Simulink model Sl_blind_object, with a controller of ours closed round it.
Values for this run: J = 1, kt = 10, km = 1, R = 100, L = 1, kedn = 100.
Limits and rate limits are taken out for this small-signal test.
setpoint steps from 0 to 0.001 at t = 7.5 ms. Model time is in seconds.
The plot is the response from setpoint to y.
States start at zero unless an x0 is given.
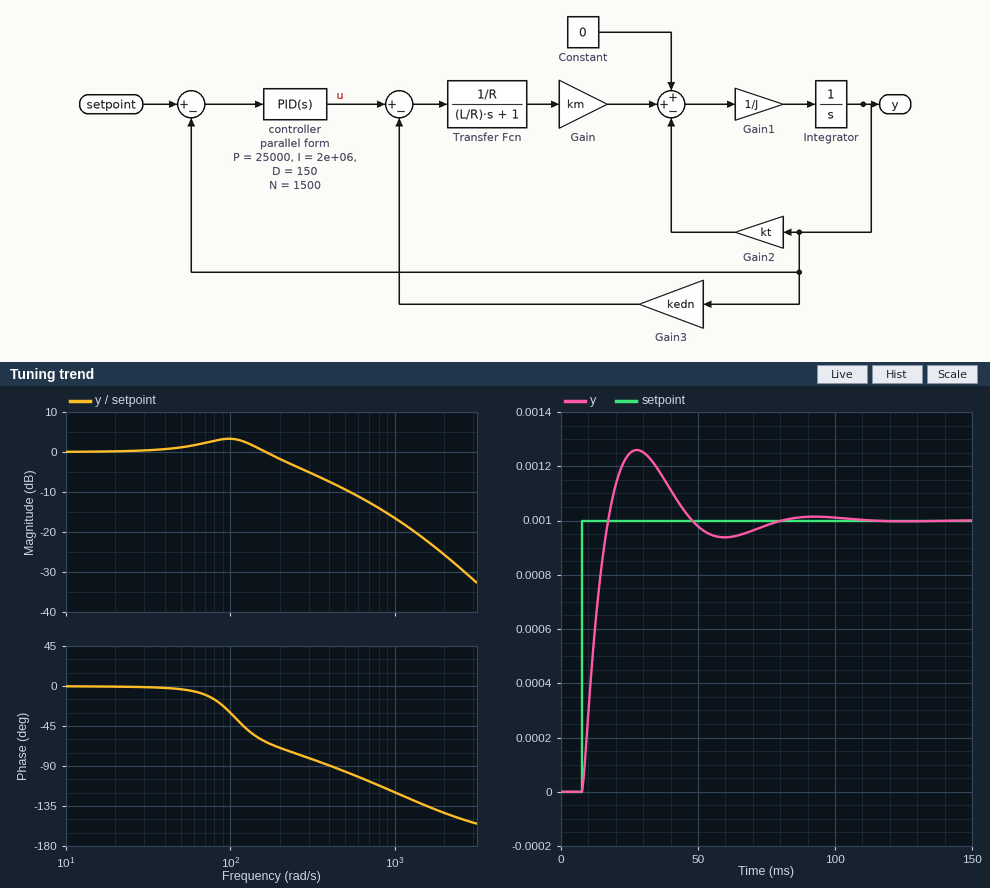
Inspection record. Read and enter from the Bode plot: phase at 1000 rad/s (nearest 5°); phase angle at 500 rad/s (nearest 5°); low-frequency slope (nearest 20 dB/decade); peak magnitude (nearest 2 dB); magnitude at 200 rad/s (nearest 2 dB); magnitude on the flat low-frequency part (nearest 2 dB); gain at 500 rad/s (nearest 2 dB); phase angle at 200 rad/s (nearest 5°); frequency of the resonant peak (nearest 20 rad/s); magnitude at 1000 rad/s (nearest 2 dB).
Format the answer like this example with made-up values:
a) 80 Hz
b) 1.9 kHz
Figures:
a) -120°
b) -95°
c) 0 dB/decade
d) 4 dB
e) -2 dB
f) 0 dB
g) -10 dB
h) -70°
i) 100 rad/s
j) -16 dB
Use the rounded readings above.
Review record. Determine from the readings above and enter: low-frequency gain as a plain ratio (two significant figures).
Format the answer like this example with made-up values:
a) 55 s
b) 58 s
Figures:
a) 1.0
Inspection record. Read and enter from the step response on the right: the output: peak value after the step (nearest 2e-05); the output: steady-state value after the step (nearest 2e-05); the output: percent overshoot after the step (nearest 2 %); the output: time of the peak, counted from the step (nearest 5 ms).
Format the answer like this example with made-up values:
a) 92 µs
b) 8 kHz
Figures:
a) 0.00126
b) 0.00100
c) 26 %
d) 20 ms
